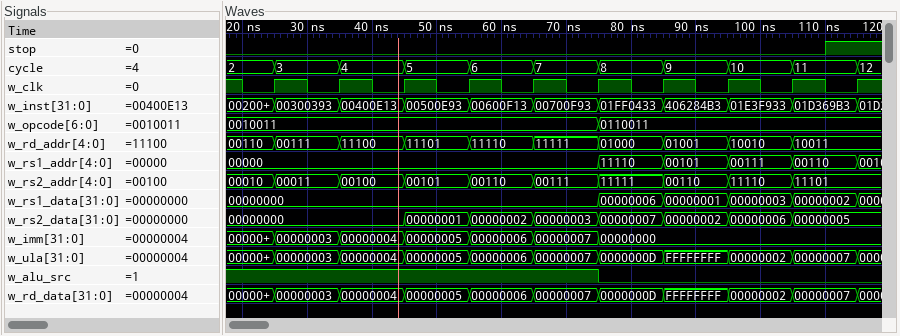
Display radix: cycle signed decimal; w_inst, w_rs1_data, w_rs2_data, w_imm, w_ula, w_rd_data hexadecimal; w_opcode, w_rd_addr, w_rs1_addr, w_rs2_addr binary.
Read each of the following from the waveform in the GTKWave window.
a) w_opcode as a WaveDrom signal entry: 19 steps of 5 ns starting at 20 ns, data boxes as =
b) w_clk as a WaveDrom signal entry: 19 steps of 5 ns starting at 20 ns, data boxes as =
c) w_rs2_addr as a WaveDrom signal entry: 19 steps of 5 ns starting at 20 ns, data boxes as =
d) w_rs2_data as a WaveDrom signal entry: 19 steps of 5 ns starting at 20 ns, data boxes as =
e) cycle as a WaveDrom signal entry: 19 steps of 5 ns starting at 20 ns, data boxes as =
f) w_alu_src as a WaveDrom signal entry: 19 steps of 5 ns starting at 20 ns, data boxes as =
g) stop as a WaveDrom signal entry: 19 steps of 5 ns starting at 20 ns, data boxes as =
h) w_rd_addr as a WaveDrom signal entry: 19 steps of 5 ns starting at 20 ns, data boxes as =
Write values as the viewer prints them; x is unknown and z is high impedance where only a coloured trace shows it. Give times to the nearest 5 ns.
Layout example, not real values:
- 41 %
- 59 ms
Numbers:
- {name: 'w_opcode', wave: '=..........=.......', data: '0010011 0110011'}
- {name: 'w_clk', wave: '0101010101010101010'}
- {name: 'w_rs2_addr', wave: '==.=.=.=.=.=.=.=.=.', data: '00010 00011 00100 00101 00110 00111 11111 00110 11110 11101'}
- {name: 'w_rs2_data', wave: '=....=.=.=.=.=.=.=.', data: '00000000 00000001 00000002 00000003 00000007 00000002 00000006 00000005'}
- {name: 'cycle', wave: '==.=.=.=.=.=.=.=.=.', data: '2 3 4 5 6 7 8 9 10 11'}
- {name: 'w_alu_src', wave: '1..........0.......'}
- {name: 'stop', wave: '0.................1'}
- {name: 'w_rd_addr', wave: '==.=.=.=.=.=.=.=.=.', data: '00110 00111 11100 11101 11110 11111 01000 01001 10010 10011'}
